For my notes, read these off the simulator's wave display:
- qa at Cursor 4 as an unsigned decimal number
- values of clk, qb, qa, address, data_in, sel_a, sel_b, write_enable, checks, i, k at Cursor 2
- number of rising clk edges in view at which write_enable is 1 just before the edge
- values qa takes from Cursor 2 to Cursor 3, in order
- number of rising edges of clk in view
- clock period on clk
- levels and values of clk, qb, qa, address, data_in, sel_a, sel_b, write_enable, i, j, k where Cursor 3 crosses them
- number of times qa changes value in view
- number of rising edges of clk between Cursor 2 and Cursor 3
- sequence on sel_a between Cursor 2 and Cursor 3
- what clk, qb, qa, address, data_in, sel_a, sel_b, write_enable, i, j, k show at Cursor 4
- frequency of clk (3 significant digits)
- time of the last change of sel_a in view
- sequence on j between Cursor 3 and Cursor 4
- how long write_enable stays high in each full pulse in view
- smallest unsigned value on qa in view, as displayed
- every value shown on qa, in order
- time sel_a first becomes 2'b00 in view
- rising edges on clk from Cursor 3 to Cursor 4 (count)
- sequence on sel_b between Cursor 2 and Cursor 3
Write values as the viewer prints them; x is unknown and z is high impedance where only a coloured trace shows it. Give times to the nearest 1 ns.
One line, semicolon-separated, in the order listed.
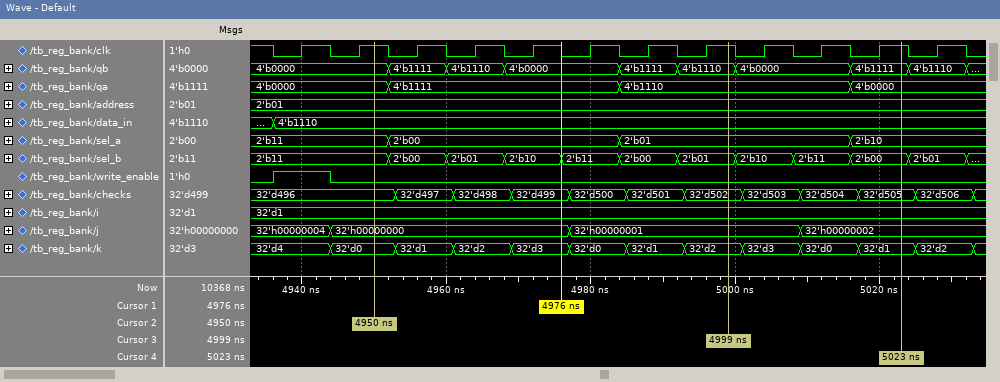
0; clk=1, qb=4'b0000, qa=4'b0000, address=2'b01, data_in=4'b1110, sel_a=2'b11, sel_b=2'b11, write_enable=0, checks=32'd496, i=32'd1, k=32'd0; 1; 4'b0000, 4'b1111, 4'b1110; 12; 8 ns; clk=1, qb=4'b1110, qa=4'b1110, address=2'b01, data_in=4'b1110, sel_a=2'b01, sel_b=2'b01, write_enable=0, i=32'd1, j=32'h00000001, k=32'd2; 3; 6; 2'b11, 2'b00, 2'b01; clk=1, qb=4'b1111, qa=4'b0000, address=2'b01, data_in=4'b1110, sel_a=2'b10, sel_b=2'b00, write_enable=0, i=32'd1, j=32'h00000002, k=32'd1; 125 MHz; 5016 ns; 32'h00000001, 32'h00000002; 8 ns; 4'b0000; 4'b0000, 4'b1111, 4'b1110, 4'b0000; 4952 ns; 3; 2'b11, 2'b00, 2'b01, 2'b10, 2'b11, 2'b00, 2'b01
